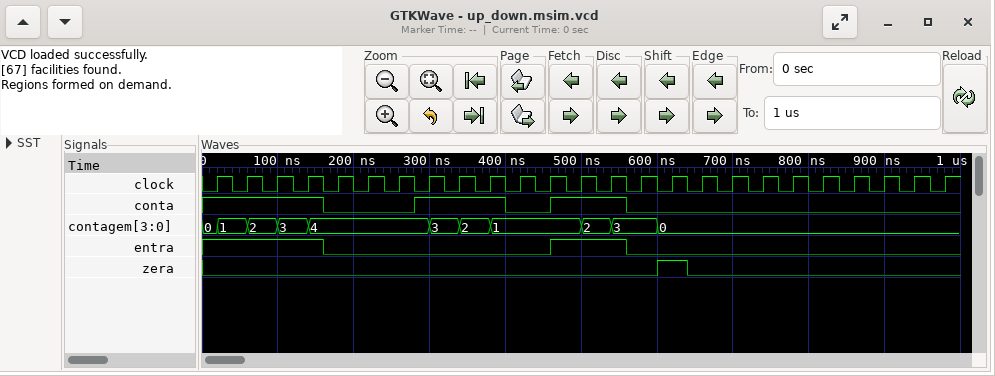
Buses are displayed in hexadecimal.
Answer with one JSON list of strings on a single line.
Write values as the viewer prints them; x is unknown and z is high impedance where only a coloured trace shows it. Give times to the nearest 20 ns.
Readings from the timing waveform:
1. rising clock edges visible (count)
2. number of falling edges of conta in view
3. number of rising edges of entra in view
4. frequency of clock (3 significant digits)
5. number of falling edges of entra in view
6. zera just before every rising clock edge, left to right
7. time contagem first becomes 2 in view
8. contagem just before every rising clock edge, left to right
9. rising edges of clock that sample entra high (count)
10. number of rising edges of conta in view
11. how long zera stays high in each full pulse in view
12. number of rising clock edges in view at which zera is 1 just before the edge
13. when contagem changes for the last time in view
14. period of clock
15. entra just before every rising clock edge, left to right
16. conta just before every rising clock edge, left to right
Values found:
["25", "3", "1", "25.0 MHz", "2", "0 0 0 0 0 0 0 0 0 0 0 0 0 0 0 1 0 0 0 0 0 0 0 0 0", "60 ns", "0, 1, 2, 3, 4, 4, 4, 4, 3, 2, 1, 1, 1, 2, 3, 0, 0, 0, 0, 0, 0, 0, 0, 0, 0", "6", "2", "40 ns", "1", "600 ns", "40 ns", "1 1 1 1 0 0 0 0 0 0 0 0 1 1 0 0 0 0 0 0 0 0 0 0 0", "1 1 1 1 0 0 0 1 1 1 0 0 1 1 0 0 0 0 0 0 0 0 0 0 0"]
